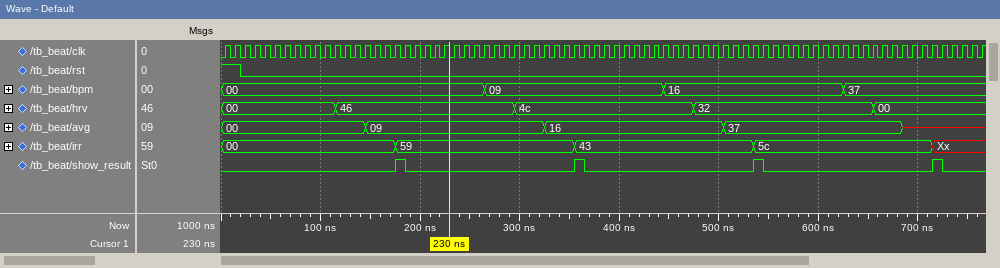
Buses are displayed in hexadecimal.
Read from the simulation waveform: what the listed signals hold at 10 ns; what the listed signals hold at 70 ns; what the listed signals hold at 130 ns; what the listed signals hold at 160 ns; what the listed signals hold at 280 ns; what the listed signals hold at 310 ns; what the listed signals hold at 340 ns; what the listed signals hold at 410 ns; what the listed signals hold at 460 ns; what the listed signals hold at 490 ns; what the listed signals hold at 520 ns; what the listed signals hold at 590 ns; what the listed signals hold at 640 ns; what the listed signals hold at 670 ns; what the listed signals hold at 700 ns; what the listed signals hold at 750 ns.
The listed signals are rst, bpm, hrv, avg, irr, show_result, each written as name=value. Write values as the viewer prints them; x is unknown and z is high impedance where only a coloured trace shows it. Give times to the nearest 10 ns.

rst=1, bpm=00, hrv=00, avg=00, irr=00, show_result=0
rst=0, bpm=00, hrv=00, avg=00, irr=00, show_result=0
rst=0, bpm=00, hrv=46, avg=00, irr=00, show_result=0
rst=0, bpm=00, hrv=46, avg=09, irr=00, show_result=0
rst=0, bpm=09, hrv=46, avg=09, irr=59, show_result=0
rst=0, bpm=09, hrv=4c, avg=09, irr=59, show_result=0
rst=0, bpm=09, hrv=4c, avg=16, irr=59, show_result=0
rst=0, bpm=09, hrv=4c, avg=16, irr=43, show_result=0
rst=0, bpm=16, hrv=4c, avg=16, irr=43, show_result=0
rst=0, bpm=16, hrv=32, avg=16, irr=43, show_result=0
rst=0, bpm=16, hrv=32, avg=37, irr=43, show_result=0
rst=0, bpm=16, hrv=32, avg=37, irr=5c, show_result=0
rst=0, bpm=37, hrv=32, avg=37, irr=5c, show_result=0
rst=0, bpm=37, hrv=00, avg=37, irr=5c, show_result=0
rst=0, bpm=37, hrv=00, avg=x, irr=5c, show_result=0
rst=0, bpm=37, hrv=00, avg=x, irr=Xx, show_result=0
